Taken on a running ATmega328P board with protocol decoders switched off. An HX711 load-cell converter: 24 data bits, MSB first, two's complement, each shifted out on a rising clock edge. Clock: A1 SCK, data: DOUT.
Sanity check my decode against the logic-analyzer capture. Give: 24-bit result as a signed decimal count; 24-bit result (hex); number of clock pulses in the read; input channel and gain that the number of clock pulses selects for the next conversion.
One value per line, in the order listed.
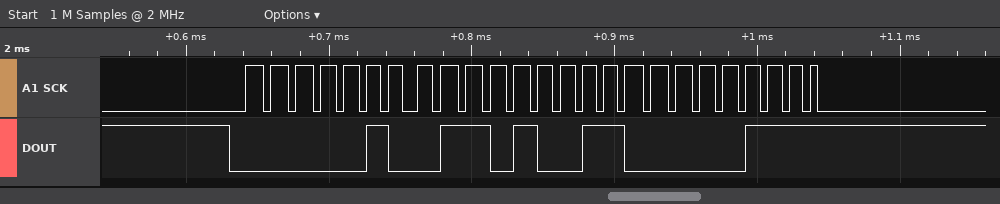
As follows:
316167
0x04D307
25
channel A, gain 128
